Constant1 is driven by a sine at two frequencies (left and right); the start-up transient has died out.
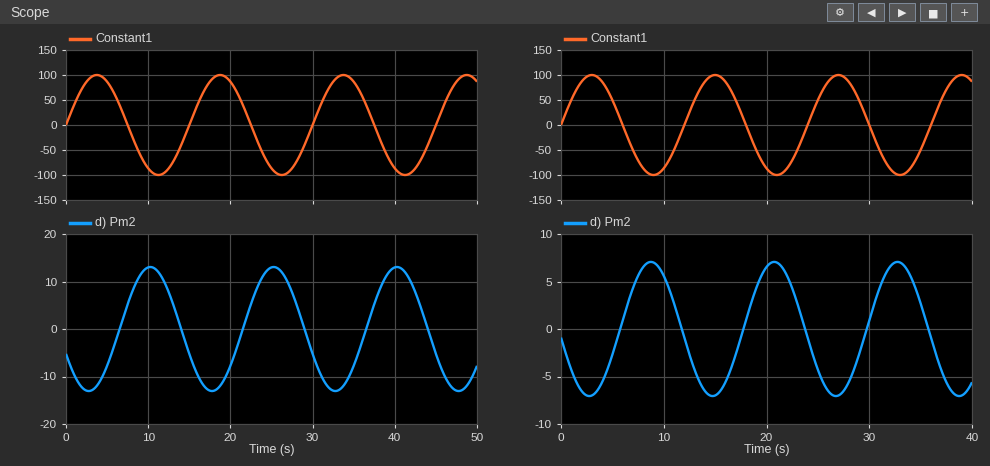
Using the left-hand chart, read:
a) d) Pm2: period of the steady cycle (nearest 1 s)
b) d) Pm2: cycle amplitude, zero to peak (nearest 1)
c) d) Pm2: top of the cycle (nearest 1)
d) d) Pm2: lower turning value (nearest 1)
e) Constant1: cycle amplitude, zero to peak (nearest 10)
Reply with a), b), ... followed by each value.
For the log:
a) 15 s
b) 13
c) 13
d) -13
e) 100
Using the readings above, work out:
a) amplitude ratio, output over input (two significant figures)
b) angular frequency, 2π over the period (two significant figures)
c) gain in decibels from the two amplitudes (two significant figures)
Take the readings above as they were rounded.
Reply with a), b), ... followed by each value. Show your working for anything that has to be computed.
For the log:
a) 13 / 100 = 0.13
b) 2π / 15 = 0.42 rad/s
c) 20 log10(13 / 100) = -18 dB
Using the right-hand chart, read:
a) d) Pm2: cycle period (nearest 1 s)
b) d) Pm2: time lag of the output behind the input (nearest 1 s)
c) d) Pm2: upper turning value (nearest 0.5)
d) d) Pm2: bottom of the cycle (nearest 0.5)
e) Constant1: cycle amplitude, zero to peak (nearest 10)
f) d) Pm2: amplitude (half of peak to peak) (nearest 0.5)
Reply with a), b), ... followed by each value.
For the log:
a) 12 s
b) 6 s
c) 7.0
d) -7.0
e) 100
f) 7.0
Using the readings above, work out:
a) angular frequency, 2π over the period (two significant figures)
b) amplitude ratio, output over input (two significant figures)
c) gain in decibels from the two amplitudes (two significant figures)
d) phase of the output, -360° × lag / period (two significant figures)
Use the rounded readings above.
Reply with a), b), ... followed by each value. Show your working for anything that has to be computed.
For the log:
a) 2π / 12 = 0.52 rad/s
b) 7 / 100 = 0.070
c) 20 log10(7 / 100) = -23 dB
d) -360 × 6 / 12 = -180°
